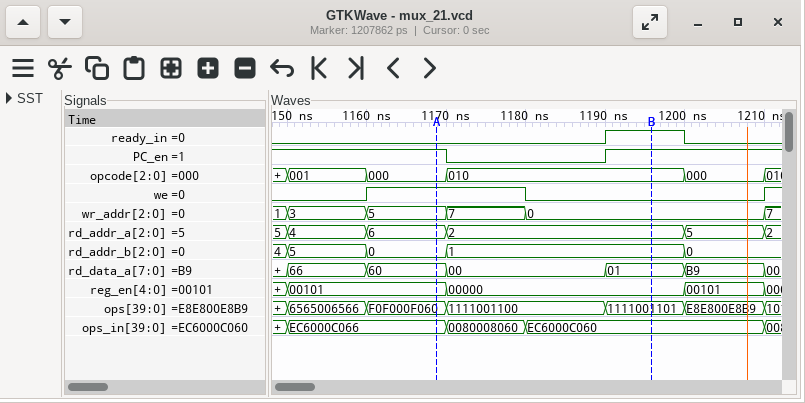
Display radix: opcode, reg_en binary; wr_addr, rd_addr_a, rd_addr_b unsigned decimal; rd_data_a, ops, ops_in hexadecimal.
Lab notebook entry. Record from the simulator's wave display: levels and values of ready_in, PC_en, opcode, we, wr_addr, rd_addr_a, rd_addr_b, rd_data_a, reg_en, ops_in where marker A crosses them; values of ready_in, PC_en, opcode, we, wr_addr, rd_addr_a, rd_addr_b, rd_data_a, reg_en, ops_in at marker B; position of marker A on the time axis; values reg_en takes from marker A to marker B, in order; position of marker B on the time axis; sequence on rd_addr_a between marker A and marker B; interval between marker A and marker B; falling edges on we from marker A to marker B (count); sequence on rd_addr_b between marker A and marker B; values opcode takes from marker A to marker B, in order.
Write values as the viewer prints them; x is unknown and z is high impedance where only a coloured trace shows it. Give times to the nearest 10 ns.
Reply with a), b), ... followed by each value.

a) ready_in=0, PC_en=1, opcode=000, we=1, wr_addr=5, rd_addr_a=6, rd_addr_b=0, rd_data_a=60, reg_en=00101, ops_in=EC6000C066
b) ready_in=1, PC_en=1, opcode=010, we=0, wr_addr=0, rd_addr_a=2, rd_addr_b=1, rd_data_a=01, reg_en=00000, ops_in=EC6000C060
c) 1170 ns
d) 00101, 00000
e) 1200 ns
f) 6, 2
g) 30 ns
h) 1
i) 0, 1
j) 000, 010
